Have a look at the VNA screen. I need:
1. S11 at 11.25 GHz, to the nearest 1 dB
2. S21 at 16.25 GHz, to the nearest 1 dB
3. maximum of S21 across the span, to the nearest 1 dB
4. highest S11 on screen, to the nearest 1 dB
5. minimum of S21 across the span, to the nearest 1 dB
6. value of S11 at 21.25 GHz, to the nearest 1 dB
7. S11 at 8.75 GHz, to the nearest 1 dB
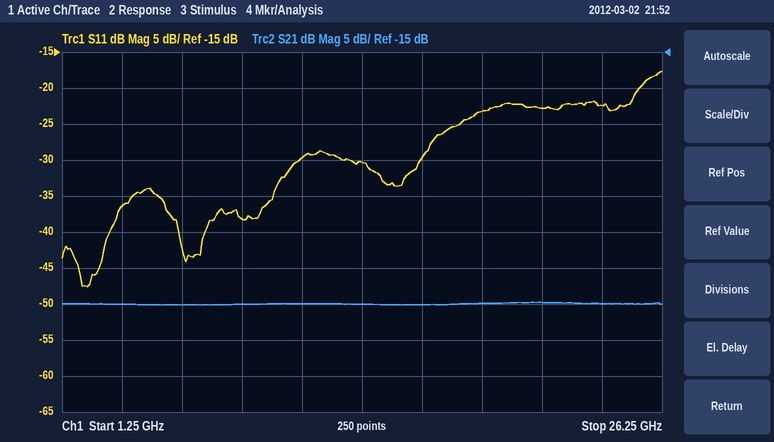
-30 dB
-50 dB
-50 dB
-18 dB
-50 dB
-23 dB
-38 dB
